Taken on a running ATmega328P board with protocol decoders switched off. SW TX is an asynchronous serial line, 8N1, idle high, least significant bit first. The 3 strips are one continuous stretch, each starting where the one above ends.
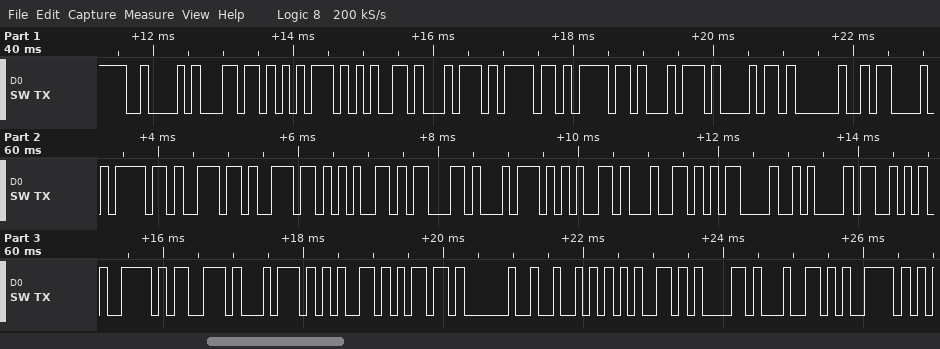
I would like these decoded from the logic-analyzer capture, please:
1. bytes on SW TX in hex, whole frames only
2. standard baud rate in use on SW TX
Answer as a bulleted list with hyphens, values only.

- 42 6C 75 65 74 6F 6F 74 68 20 43 6F 6E 6E 65 63 74 65 64 0D 0A 53 79 73 74 65 6D 20 52 65 61 64 79
- 9600 baud
